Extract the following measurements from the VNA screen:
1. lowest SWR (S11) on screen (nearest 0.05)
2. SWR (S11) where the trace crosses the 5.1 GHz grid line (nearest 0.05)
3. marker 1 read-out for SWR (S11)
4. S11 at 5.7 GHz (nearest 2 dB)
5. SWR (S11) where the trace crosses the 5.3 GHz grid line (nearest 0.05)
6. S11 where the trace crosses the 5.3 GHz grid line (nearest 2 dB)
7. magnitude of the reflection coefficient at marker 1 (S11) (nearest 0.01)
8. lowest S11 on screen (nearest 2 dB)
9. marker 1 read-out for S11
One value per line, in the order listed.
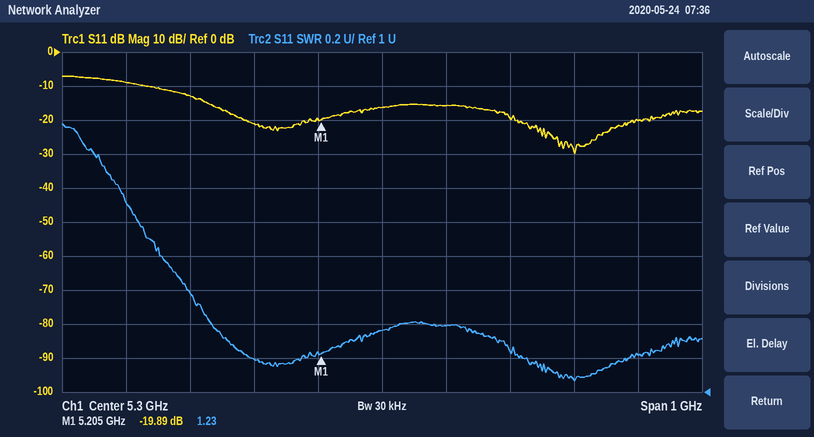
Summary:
1.05
1.20
1.23
-20 dB
1.35
-16 dB
0.10
-30 dB
-19.89 dB
